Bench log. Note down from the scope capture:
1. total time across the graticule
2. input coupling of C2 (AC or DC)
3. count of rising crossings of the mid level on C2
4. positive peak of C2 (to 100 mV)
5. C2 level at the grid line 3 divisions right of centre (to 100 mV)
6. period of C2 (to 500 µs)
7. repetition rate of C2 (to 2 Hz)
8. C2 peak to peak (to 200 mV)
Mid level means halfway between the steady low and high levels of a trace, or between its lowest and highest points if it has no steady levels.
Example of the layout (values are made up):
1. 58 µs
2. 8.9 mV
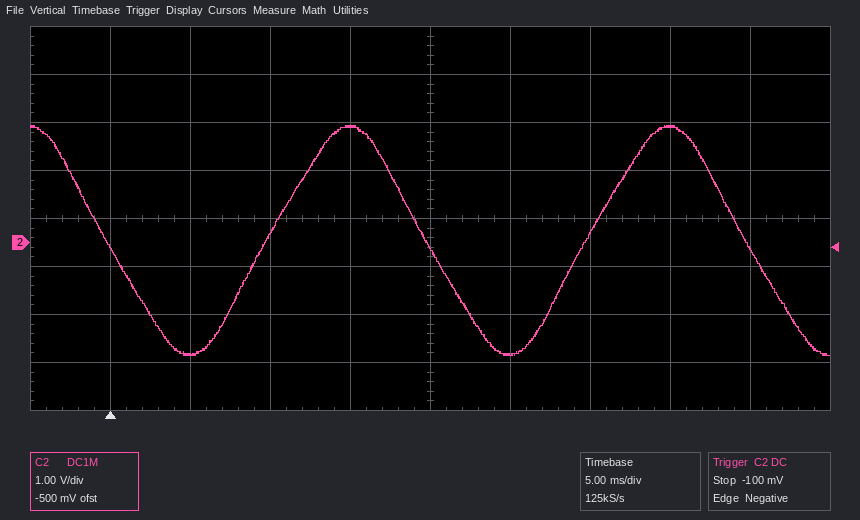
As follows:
1. 50 ms
2. DC
3. 2
4. 2.4 V
5. 2.4 V
6. 20.0 ms
7. 50 Hz
8. 4.8 V
